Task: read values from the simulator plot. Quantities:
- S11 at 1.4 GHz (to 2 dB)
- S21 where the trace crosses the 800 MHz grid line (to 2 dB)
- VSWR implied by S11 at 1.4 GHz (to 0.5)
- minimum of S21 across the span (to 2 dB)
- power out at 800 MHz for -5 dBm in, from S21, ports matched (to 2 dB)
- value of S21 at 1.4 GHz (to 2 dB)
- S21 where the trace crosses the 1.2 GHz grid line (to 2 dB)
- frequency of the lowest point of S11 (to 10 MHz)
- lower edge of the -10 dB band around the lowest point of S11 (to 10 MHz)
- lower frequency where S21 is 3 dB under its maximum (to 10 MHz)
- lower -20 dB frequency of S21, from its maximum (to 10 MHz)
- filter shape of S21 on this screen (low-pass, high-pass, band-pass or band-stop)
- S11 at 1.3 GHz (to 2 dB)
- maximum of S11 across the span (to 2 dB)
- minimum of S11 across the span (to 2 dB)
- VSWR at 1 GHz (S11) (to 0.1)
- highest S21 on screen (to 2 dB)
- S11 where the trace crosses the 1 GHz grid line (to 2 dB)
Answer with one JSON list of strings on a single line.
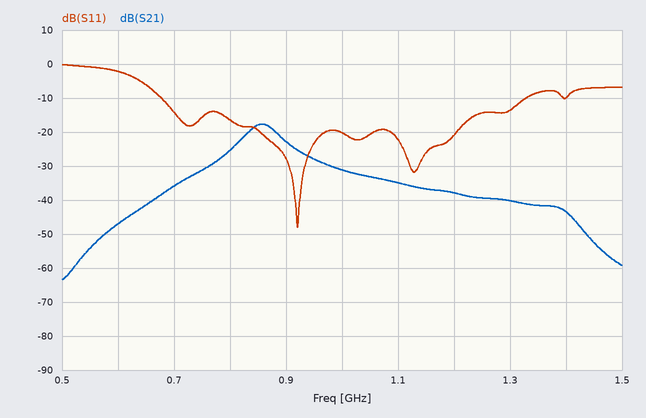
["-10 dB", "-26 dB", "2.0", "-64 dB", "-30 dBm", "-44 dB", "-38 dB", "920 MHz", "680 MHz", "830 MHz", "680 MHz", "band-pass", "-14 dB", "0 dB", "-48 dB", "1.2", "-18 dB", "-20 dB"]
